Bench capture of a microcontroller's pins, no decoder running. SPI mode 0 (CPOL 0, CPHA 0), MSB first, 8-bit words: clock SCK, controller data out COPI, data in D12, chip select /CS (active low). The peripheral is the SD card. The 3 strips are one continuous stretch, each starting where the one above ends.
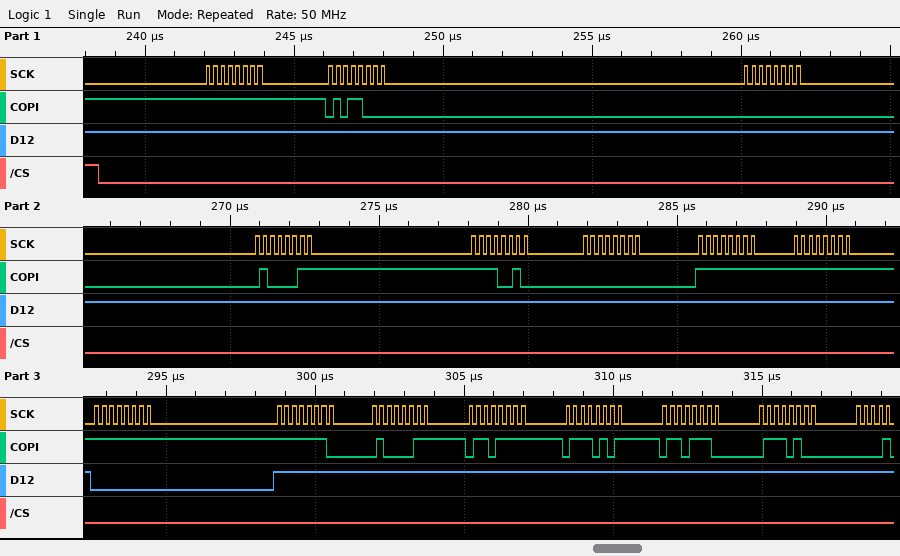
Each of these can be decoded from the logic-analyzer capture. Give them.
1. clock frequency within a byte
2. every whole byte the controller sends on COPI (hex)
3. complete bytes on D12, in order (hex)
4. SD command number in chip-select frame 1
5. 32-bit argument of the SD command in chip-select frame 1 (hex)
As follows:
4 MHz
FF 58 00 43 F2 00 FF FF FF FE 43 6F 75 6E 74
FF FF FF FF FF FF FF FF 00 FF FF FF FF FF FF
CMD24
0x0043F200
